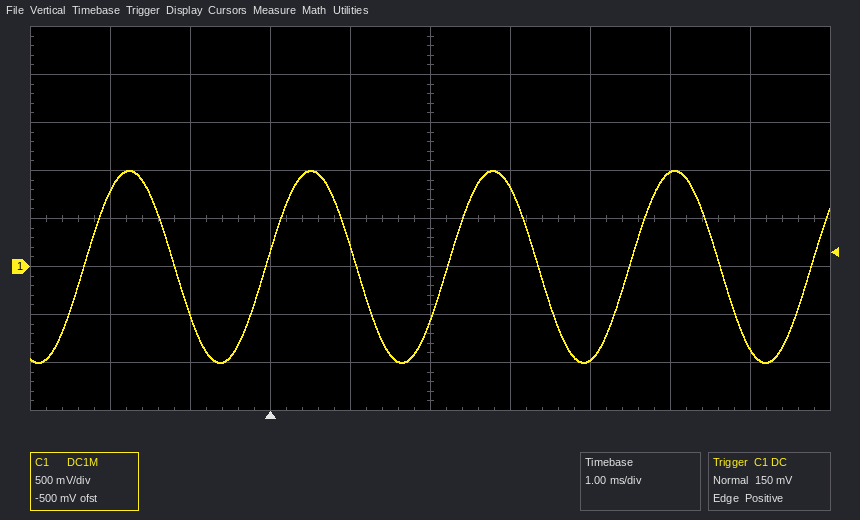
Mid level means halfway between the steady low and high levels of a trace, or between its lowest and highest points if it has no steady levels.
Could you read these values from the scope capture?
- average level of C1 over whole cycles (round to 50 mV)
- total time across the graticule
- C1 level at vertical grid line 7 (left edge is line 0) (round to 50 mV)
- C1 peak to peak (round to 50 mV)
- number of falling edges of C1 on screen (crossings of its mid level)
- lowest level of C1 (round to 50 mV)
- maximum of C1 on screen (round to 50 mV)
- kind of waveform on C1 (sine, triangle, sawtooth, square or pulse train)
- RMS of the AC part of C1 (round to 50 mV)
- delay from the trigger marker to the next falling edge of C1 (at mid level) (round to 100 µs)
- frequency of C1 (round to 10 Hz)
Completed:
0 mV
10 ms
-950 mV
2.00 V
4
-1.00 V
1.00 V
sine
700 mV
1.1 ms
440 Hz
